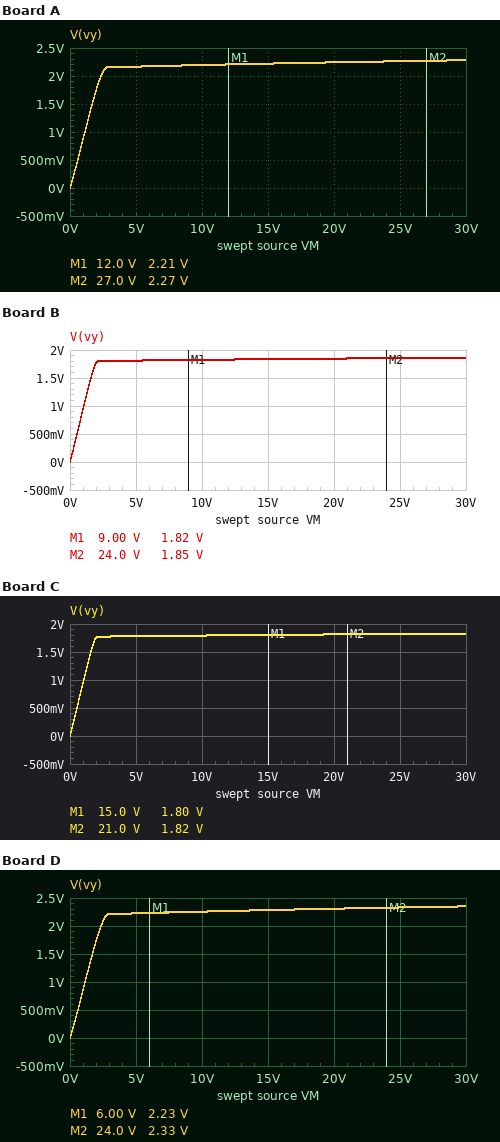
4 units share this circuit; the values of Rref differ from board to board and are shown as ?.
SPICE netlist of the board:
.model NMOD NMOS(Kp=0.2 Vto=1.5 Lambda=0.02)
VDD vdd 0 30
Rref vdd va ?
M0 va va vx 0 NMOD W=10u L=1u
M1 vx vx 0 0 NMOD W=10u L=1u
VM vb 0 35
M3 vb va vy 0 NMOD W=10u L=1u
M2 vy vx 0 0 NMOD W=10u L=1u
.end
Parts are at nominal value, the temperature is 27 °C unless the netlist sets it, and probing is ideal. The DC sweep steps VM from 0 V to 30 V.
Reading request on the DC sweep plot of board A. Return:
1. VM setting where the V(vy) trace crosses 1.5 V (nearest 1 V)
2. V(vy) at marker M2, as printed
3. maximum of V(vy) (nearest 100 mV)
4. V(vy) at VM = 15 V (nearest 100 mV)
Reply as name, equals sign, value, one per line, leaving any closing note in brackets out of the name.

VM setting where the V(vy) trace crosses 1.5 V = 2 V
V(vy) at marker M2, as printed = 2.27 V
maximum of V(vy) = 2.3 V
V(vy) at VM = 15 V = 2.2 V
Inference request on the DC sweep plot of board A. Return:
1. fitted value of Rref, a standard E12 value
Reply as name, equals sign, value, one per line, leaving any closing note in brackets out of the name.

fitted value of Rref, a standard E12 value = 56 Ω
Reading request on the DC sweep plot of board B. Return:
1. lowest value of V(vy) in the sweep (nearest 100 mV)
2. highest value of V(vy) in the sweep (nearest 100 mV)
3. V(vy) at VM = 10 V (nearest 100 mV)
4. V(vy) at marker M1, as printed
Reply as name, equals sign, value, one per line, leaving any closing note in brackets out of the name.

lowest value of V(vy) in the sweep = 0 V
highest value of V(vy) in the sweep = 1.9 V
V(vy) at VM = 10 V = 1.8 V
V(vy) at marker M1, as printed = 1.82 V
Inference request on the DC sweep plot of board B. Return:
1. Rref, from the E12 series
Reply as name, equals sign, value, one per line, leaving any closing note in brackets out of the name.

Rref, from the E12 series = 270 Ω
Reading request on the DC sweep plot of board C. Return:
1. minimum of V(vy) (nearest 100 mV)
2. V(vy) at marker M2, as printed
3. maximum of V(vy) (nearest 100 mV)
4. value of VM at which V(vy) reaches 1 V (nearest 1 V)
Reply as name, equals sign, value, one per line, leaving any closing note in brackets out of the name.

minimum of V(vy) = 0 V
V(vy) at marker M2, as printed = 1.82 V
maximum of V(vy) = 1.8 V
value of VM at which V(vy) reaches 1 V = 1 V
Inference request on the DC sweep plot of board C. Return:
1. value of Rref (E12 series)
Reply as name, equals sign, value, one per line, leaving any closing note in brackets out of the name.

value of Rref = 330 Ω
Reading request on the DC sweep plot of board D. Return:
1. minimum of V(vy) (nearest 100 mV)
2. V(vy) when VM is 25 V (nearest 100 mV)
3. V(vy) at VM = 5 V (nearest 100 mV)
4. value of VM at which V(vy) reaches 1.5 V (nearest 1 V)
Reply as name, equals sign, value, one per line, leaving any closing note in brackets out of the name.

minimum of V(vy) = 0 V
V(vy) when VM is 25 V = 2.3 V
V(vy) at VM = 5 V = 2.2 V
value of VM at which V(vy) reaches 1.5 V = 2 V
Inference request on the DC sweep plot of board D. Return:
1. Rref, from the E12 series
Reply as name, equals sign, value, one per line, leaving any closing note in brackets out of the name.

Rref, from the E12 series = 47 Ω
